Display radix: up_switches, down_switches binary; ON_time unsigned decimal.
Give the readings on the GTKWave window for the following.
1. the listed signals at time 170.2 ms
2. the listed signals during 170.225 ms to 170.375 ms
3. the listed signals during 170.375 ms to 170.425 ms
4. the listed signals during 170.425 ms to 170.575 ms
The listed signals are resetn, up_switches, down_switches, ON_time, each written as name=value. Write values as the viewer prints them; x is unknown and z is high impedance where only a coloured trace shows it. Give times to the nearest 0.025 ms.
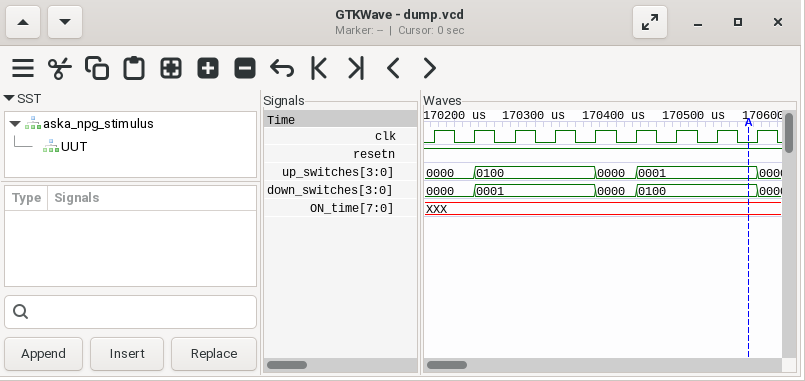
resetn=1, up_switches=0000, down_switches=0000, ON_time=XXX
resetn=1, up_switches=0100, down_switches=0001, ON_time=XXX
resetn=1, up_switches=0000, down_switches=0000, ON_time=XXX
resetn=1, up_switches=0001, down_switches=0100, ON_time=XXX
